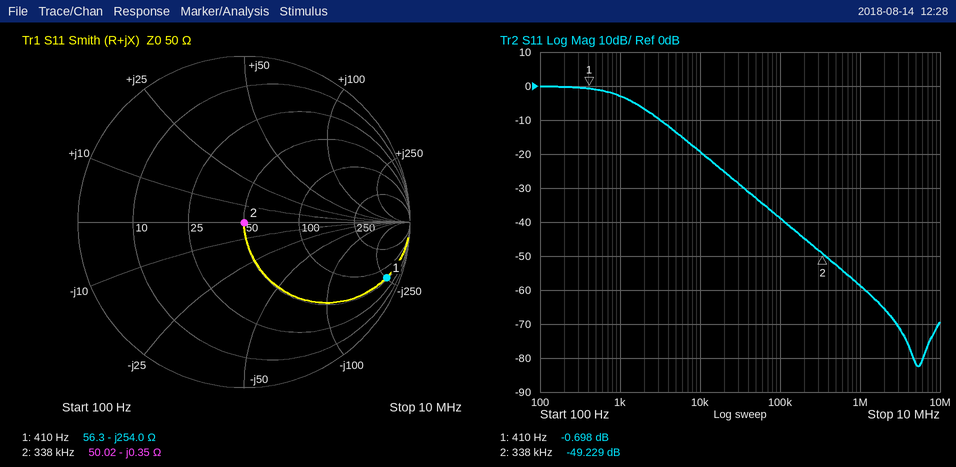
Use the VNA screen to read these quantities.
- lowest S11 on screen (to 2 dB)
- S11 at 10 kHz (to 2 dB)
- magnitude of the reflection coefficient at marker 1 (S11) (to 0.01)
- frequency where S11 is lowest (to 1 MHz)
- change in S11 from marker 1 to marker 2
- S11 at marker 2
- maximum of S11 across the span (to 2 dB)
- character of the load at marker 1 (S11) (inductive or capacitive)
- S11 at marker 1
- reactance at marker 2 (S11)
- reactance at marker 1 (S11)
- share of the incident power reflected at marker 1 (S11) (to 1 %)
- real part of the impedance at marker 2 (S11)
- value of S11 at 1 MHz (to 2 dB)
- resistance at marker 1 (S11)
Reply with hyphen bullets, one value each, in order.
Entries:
- -82 dB
- -20 dB
- 0.92
- 5 MHz
- -48.531 dB
- -49.229 dB
- 0 dB
- capacitive
- -0.698 dB
- -0.35 Ω
- -254.0 Ω
- 85 %
- 50.02 Ω
- -58 dB
- 56.3 Ω
